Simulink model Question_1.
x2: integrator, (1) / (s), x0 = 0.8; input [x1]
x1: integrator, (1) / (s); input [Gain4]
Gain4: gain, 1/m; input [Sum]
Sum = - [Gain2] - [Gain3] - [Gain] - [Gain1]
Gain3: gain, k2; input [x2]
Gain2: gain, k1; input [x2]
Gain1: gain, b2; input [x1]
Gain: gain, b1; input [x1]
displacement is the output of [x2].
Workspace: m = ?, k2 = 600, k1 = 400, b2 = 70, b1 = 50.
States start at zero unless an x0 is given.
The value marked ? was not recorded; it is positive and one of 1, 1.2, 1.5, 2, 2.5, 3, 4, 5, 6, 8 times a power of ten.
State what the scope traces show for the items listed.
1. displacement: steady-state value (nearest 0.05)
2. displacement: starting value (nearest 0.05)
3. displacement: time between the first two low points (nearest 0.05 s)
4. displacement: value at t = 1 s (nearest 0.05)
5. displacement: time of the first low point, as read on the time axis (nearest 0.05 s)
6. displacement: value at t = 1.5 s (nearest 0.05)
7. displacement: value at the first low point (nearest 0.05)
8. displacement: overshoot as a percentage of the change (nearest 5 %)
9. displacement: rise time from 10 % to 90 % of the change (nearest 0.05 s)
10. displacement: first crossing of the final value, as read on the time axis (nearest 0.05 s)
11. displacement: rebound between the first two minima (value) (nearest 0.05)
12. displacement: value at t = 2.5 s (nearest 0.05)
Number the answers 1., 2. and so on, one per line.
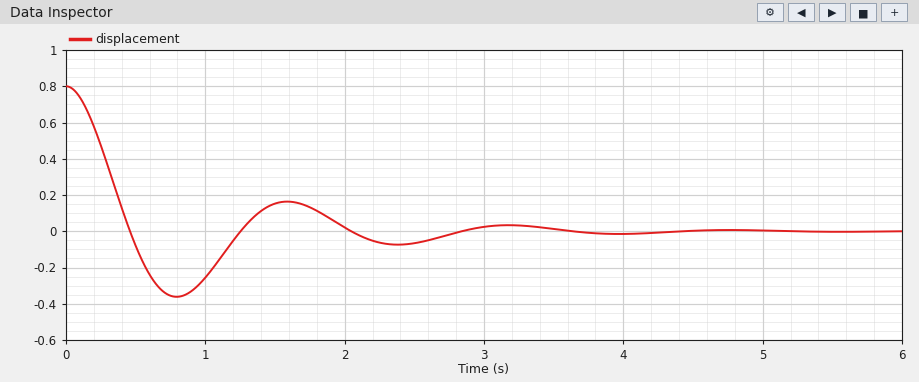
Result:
1. 0.00
2. 0.80
3. 1.60 s
4. -0.25
5. 0.80 s
6. 0.15
7. -0.35
8. 45 %
9. 0.30 s
10. 0.45 s
11. 0.15
12. -0.05
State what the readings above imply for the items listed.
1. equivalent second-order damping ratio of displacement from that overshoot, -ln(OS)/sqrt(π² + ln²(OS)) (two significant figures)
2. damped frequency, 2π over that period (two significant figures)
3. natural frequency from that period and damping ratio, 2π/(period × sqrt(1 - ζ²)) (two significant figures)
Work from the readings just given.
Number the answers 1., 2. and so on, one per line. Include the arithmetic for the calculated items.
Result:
1. ln(0.45) = -0.799; 0.799 / sqrt(9.870 + 0.638) = 0.25
2. 2π / 1.6 = 3.9 rad/s
3. 2π / (1.6 × sqrt(1 - 0.25²)) = 4.1 rad/s
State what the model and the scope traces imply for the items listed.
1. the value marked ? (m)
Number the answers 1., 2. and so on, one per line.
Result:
1. 60
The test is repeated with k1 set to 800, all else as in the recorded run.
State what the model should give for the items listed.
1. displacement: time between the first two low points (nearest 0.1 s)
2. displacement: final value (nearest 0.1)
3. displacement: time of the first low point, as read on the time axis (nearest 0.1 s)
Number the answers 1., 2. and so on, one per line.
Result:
1. 1.3 s
2. 0.0
3. 0.7 s
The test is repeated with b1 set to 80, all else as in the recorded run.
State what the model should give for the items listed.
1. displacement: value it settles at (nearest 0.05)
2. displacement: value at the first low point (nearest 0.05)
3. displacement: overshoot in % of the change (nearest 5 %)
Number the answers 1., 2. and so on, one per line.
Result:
1. 0.00
2. -0.30
3. 35 %
